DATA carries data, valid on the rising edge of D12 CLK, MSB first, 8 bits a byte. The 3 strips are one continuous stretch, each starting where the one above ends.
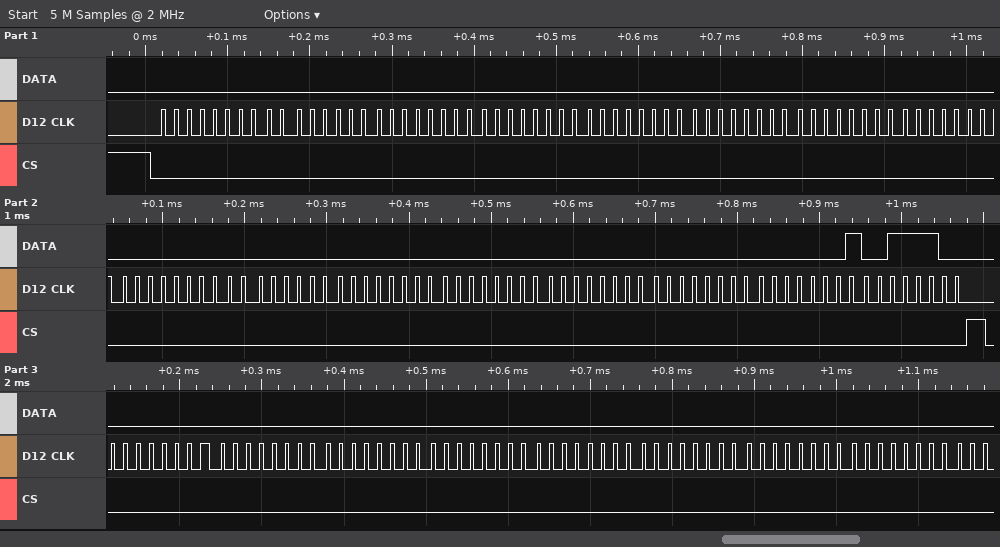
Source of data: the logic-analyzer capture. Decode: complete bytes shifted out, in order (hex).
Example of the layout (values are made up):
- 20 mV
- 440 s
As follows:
- 0x00 0x00 0x00 0x00 0x00 0x00 0x00 0x00 0x00 0x00 0x00 0x00 0x00 0x00 0x01 0x3C 0x00 0x00 0x00 0x00 0x00 0x00 0x00 0x00
